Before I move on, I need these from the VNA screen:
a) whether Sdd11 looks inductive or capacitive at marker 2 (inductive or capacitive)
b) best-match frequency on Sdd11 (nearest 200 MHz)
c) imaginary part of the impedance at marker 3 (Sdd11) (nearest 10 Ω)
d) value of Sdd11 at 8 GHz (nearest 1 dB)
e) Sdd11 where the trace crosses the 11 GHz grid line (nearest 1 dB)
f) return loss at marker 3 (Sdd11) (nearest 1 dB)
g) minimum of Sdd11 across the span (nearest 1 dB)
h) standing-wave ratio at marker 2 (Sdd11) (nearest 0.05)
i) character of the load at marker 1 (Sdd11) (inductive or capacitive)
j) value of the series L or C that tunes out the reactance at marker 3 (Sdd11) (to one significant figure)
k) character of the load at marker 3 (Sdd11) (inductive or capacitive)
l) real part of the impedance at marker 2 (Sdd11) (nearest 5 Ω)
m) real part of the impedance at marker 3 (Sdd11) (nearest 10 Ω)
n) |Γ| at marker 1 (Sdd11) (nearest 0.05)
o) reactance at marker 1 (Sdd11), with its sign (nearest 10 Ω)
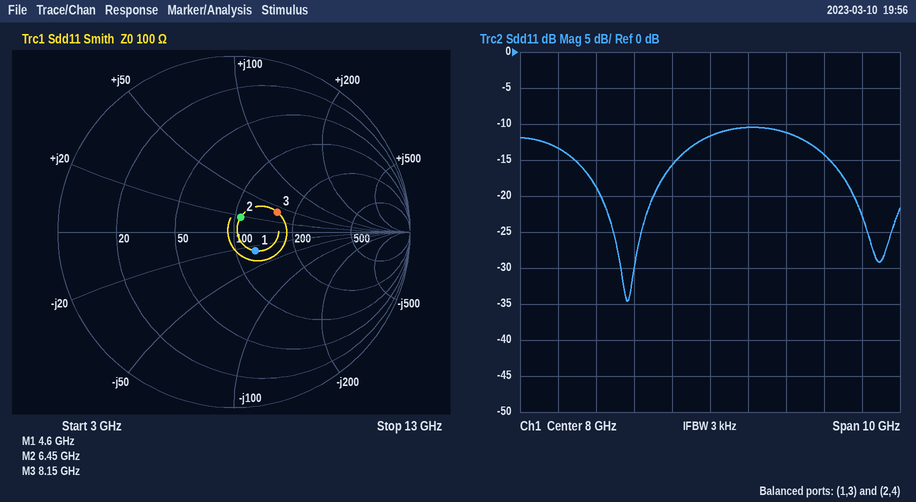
inductive
5.8 GHz
+40 Ω
-12 dB
-14 dB
11 dB
-35 dB
1.20
capacitive
500 fF
inductive
105 Ω
160 Ω
0.15
-30 Ω
